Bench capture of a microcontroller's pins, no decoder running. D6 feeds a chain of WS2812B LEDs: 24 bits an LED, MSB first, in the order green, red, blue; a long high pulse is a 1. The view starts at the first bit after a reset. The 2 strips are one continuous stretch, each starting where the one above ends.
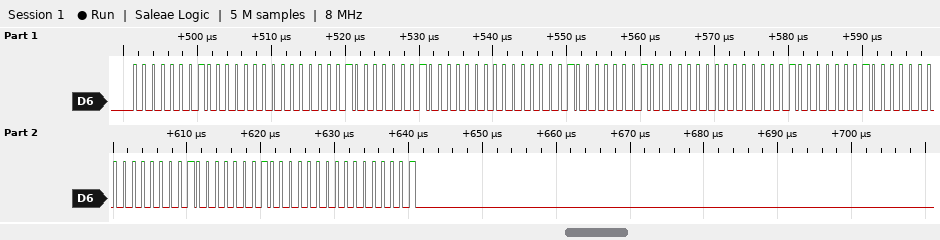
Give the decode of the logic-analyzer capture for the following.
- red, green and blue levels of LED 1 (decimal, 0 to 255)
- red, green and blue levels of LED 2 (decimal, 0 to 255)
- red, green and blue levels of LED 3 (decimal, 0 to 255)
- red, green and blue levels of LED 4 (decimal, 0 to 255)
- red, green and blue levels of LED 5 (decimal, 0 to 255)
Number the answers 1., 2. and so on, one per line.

1. 0, 1, 1
2. 0, 1, 1
3. 0, 1, 1
4. 0, 1, 1
5. 0, 1, 1
